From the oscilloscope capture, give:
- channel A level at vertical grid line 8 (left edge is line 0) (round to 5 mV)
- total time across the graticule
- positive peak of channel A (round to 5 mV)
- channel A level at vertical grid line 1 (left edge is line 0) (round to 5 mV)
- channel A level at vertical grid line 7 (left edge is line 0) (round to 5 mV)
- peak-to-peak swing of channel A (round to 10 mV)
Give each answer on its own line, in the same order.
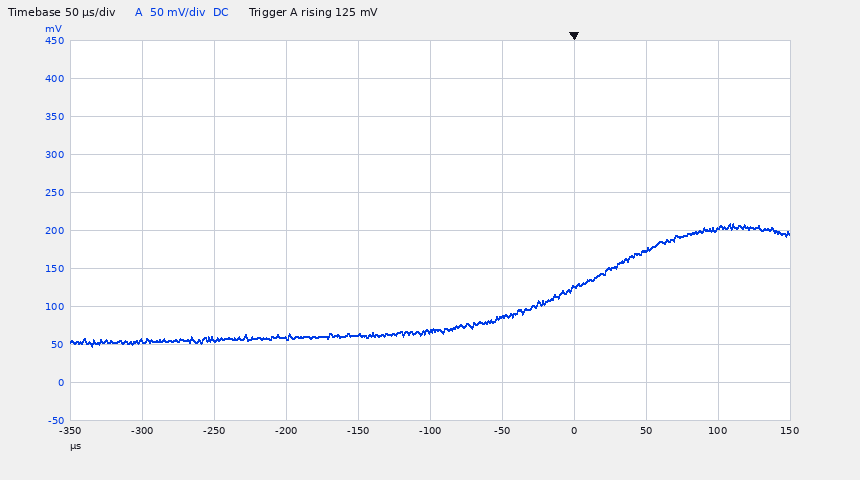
175 mV
500 µs
210 mV
55 mV
125 mV
160 mV
